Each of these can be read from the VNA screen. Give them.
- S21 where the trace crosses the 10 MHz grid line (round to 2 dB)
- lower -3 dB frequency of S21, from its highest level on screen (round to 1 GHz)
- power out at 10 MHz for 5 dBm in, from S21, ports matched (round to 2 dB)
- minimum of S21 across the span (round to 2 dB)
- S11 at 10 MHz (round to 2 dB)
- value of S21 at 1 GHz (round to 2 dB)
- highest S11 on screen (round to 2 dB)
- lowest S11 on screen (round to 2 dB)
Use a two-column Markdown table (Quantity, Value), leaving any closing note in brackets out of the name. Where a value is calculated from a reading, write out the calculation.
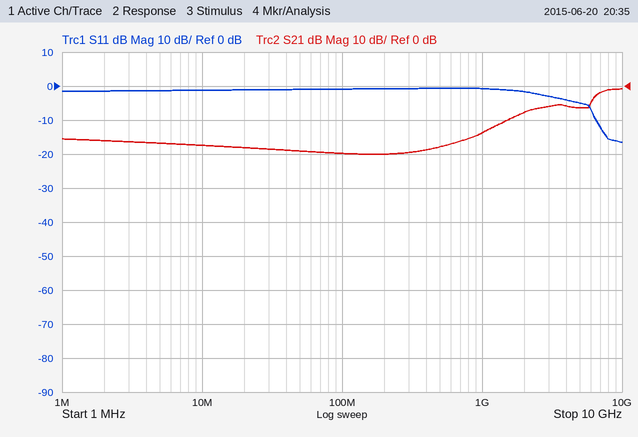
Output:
| Quantity | Value |
|---|---|
| S21 where the trace crosses the 10 MHz grid line | -18 dB |
| lower -3 dB frequency of S21, from its highest level on screen | 6 GHz |
| power out at 10 MHz for 5 dBm in, from S21, ports matched | 5 dBm + (-18 dB) = -12 dBm |
| minimum of S21 across the span | -20 dB |
| S11 at 10 MHz | -2 dB |
| value of S21 at 1 GHz | -14 dB |
| highest S11 on screen | 0 dB |
| lowest S11 on screen | -16 dB |
